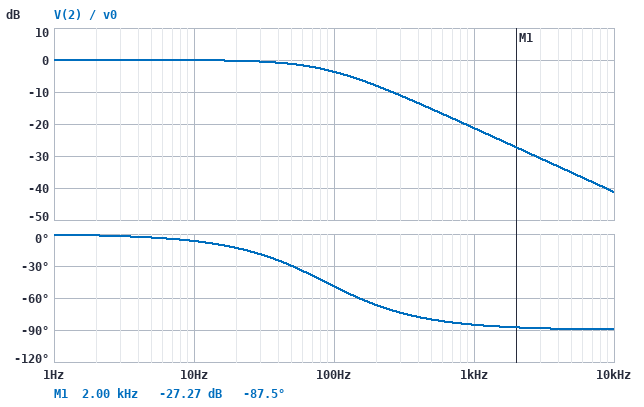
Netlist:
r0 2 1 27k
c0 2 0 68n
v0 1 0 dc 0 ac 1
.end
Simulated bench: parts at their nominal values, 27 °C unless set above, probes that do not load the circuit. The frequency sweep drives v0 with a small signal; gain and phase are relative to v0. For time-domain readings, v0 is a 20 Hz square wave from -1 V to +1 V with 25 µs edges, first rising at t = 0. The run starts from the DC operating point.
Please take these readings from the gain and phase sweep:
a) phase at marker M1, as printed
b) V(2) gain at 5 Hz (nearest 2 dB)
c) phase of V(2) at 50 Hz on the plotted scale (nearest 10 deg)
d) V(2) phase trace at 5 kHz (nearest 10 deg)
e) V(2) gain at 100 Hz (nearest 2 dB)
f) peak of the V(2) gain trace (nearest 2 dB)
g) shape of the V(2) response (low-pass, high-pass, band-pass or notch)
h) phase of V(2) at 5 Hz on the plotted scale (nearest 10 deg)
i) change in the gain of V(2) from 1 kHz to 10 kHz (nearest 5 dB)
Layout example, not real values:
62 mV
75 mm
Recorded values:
-87.5 deg
0 dB
-30 deg
-90 deg
-4 dB
0 dB
low-pass
0 deg
-20 dB
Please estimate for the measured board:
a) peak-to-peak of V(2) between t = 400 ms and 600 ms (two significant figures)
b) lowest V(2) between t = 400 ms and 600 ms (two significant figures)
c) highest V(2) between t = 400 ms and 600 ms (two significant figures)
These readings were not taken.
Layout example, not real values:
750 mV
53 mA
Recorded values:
2.0 V
-1.0 V
1.0 V
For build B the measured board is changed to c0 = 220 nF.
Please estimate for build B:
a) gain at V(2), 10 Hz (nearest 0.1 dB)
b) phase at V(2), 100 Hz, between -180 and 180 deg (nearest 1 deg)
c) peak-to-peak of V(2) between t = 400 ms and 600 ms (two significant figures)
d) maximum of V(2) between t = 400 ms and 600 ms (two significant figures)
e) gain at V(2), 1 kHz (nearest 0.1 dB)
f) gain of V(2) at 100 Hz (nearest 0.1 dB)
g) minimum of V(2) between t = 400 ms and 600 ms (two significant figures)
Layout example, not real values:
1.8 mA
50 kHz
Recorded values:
-0.6 dB
-75 deg
1.9 V
970 mV
-31.4 dB
-11.7 dB
-970 mV
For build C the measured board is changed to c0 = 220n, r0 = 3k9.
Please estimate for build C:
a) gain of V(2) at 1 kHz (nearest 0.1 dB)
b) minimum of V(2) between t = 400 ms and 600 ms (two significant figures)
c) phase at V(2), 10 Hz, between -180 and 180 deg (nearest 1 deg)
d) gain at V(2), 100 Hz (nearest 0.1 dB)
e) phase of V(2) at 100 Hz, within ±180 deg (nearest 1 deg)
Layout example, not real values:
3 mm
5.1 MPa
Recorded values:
-14.8 dB
-1.0 V
-3 deg
-1.1 dB
-28 deg
